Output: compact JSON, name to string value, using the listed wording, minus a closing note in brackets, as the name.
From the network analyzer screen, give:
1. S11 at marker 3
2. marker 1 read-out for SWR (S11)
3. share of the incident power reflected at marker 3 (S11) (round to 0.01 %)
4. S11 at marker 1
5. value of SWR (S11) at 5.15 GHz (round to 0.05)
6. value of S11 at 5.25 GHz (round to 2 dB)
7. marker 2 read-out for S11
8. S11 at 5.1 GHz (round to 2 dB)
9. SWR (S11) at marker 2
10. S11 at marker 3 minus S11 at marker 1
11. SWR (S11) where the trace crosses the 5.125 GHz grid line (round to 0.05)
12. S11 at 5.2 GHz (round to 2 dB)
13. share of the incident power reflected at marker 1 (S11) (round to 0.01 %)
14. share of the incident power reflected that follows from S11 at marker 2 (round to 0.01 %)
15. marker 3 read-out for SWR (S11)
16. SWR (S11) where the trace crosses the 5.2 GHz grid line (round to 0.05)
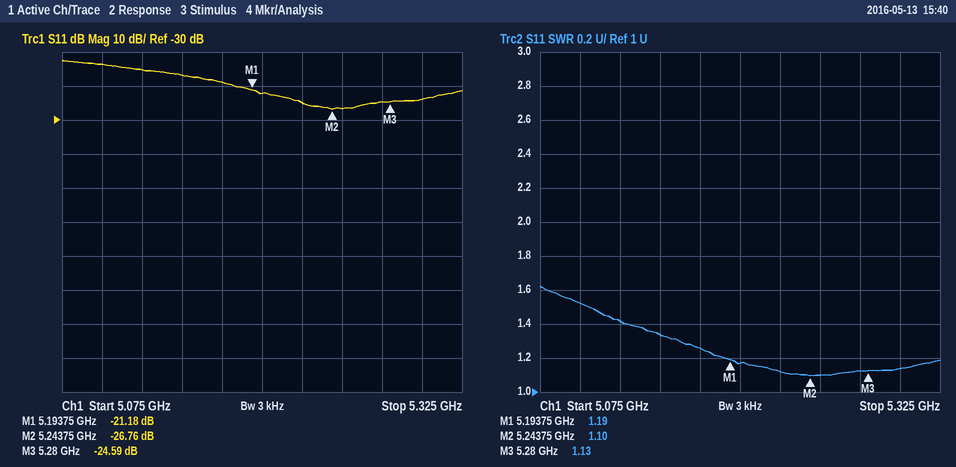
{"S11 at marker 3": "-24.59 dB", "marker 1 read-out for SWR": "1.19", "share of the incident power reflected at marker 3 (S11)": "0.35 %", "S11 at marker 1": "-21.18 dB", "value of SWR (S11) at 5.15 GHz": "1.35", "value of S11 at 5.25 GHz": "-26 dB", "marker 2 read-out for S11": "-26.76 dB", "S11 at 5.1 GHz": "-14 dB", "SWR (S11) at marker 2": "1.10", "S11 at marker 3 minus S11 at marker 1": "-3.41 dB", "SWR (S11) where the trace crosses the 5.125 GHz grid line": "1.40", "S11 at 5.2 GHz": "-22 dB", "share of the incident power reflected at marker 1 (S11)": "0.76 %", "share of the incident power reflected that follows from S11 at marker 2": "0.21 %", "marker 3 read-out for SWR": "1.13", "SWR (S11) where the trace crosses the 5.2 GHz grid line": "1.15"}
